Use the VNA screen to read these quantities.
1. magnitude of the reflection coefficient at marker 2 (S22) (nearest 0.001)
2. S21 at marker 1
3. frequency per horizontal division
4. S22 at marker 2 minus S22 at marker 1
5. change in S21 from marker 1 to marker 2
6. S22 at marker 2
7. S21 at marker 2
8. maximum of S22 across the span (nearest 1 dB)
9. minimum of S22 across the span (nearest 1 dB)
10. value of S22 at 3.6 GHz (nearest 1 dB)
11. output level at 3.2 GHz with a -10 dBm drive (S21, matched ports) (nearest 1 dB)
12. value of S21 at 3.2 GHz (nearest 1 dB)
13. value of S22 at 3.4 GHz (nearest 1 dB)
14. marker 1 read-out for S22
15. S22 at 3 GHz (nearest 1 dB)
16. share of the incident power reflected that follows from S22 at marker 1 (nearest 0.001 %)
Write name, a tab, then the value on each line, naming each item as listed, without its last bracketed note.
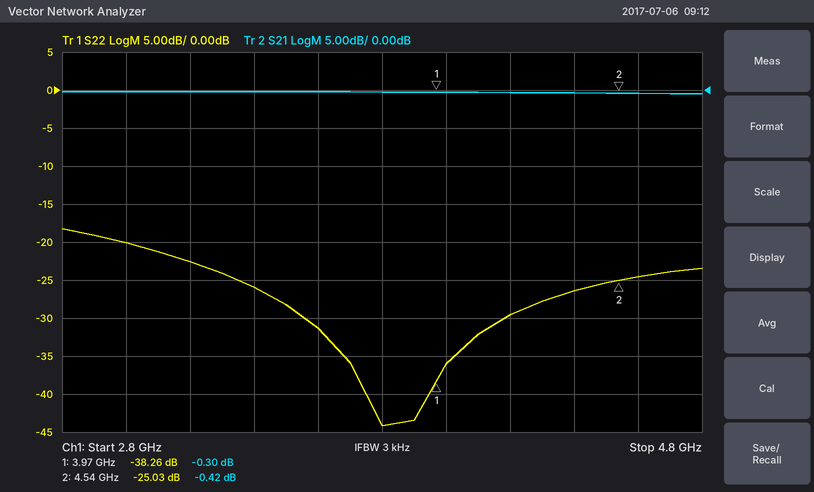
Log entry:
magnitude of the reflection coefficient at marker 2 (S22)	0.056
S21 at marker 1	-0.30 dB
frequency per horizontal division	200 MHz
S22 at marker 2 minus S22 at marker 1	13.23 dB
change in S21 from marker 1 to marker 2	-0.12 dB
S22 at marker 2	-25.03 dB
S21 at marker 2	-0.42 dB
maximum of S22 across the span	-18 dB
minimum of S22 across the span	-44 dB
value of S22 at 3.6 GHz	-31 dB
output level at 3.2 GHz with a -10 dBm drive (S21, matched ports)	-10 dBm
value of S21 at 3.2 GHz	0 dB
value of S22 at 3.4 GHz	-26 dB
marker 1 read-out for S22	-38.26 dB
S22 at 3 GHz	-20 dB
share of the incident power reflected that follows from S22 at marker 1	0.015 %
